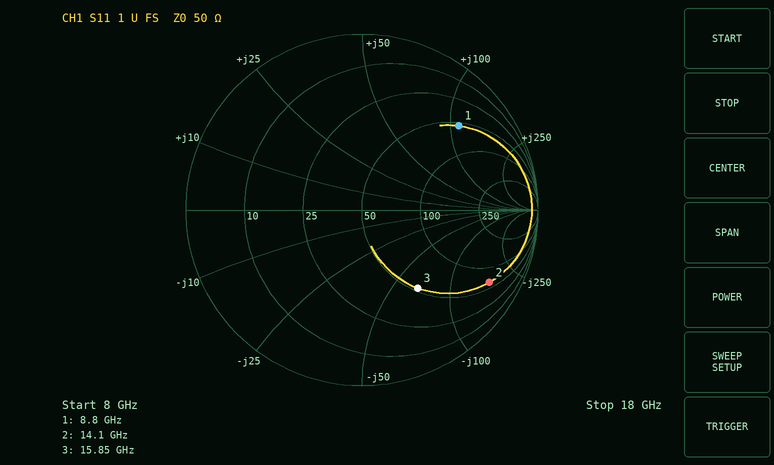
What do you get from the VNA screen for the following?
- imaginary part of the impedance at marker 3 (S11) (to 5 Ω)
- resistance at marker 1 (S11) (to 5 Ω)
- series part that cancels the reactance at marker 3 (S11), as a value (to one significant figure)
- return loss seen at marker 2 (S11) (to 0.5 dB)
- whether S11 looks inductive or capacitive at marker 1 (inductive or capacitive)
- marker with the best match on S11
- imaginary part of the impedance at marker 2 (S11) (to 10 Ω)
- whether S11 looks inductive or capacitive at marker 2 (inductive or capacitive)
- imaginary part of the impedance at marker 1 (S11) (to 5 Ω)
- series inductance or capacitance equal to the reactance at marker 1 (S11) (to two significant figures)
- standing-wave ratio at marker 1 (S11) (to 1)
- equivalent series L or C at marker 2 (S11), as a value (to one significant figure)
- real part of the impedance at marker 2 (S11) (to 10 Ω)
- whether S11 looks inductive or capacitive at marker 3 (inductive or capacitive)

-65 Ω
55 Ω
700 pH
1.5 dB
inductive
marker 3
-170 Ω
capacitive
+110 Ω
2.0 nH
6
70 fF
60 Ω
capacitive
